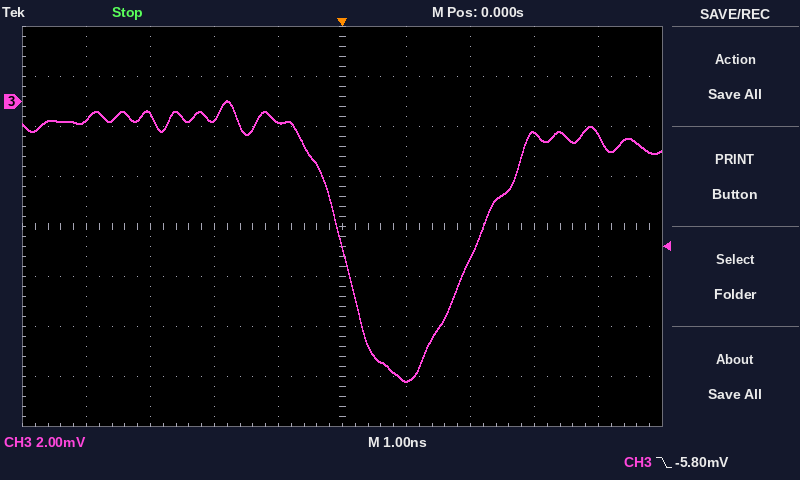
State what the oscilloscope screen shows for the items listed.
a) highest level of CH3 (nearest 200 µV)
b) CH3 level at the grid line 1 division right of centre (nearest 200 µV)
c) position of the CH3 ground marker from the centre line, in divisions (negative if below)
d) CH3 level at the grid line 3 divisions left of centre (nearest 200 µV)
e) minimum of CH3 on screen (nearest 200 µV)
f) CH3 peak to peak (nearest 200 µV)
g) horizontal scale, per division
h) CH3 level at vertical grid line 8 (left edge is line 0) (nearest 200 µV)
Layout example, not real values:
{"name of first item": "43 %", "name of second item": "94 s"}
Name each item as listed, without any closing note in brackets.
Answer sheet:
{"highest level of CH3": "0.0 mV", "CH3 level at the grid line 1 division right of centre": "-11.2 mV", "position of the CH3 ground marker from the centre line, in divisions": "+2.5 div", "CH3 level at the grid line 3 divisions left of centre": "-600 µV", "minimum of CH3 on screen": "-11.2 mV", "CH3 peak to peak": "11.2 mV", "horizontal scale, per division": "1 ns", "CH3 level at vertical grid line 8 (left edge is line 0)": "-1.2 mV"}
